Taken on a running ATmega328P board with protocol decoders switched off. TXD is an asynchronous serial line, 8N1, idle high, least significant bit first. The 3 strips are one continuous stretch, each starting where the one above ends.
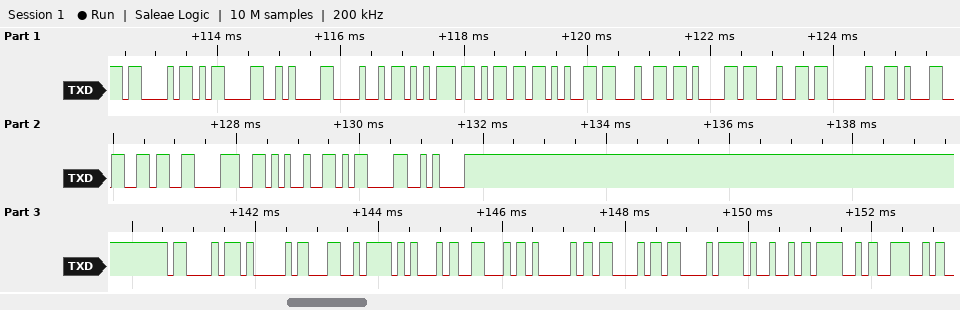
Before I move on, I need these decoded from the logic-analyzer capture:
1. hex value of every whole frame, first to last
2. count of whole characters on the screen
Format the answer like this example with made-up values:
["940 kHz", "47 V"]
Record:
["43 0D 0A 48 75 6D 65 64 61 64 20 31 36 38 25 0D 0A 43 41 4C 45 46 41 43 43 49 4F 4E", "28"]
